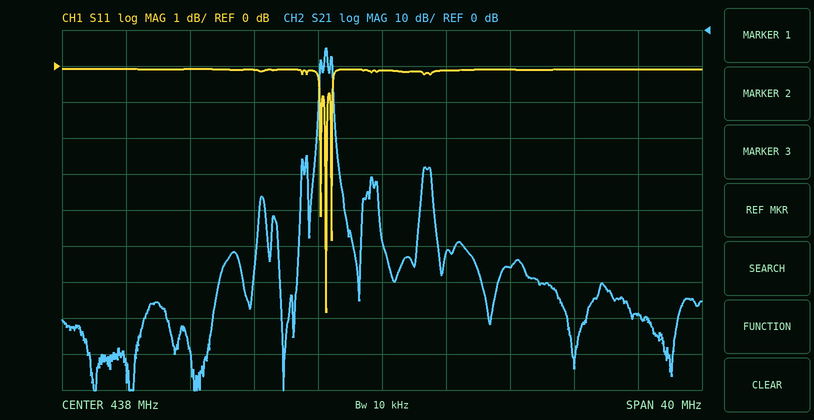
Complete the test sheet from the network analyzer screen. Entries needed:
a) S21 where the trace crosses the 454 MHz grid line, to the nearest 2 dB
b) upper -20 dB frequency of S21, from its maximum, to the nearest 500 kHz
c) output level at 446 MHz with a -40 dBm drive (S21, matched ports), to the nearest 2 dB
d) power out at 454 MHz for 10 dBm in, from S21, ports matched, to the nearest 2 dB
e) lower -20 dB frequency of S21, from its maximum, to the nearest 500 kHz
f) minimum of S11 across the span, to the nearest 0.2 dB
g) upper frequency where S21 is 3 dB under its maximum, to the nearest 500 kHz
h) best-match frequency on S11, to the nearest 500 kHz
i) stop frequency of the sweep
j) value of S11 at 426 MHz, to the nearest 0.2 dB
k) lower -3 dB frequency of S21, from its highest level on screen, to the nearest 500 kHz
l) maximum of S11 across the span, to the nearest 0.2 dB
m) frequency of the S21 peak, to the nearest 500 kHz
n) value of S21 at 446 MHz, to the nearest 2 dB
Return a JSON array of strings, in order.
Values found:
["-78 dB", "435.0 MHz", "-106 dBm", "-68 dBm", "434.0 MHz", "-6.8 dB", "434.5 MHz", "434.5 MHz", "458 MHz", "0.0 dB", "434.5 MHz", "0.0 dB", "434.5 MHz", "-66 dB"]
